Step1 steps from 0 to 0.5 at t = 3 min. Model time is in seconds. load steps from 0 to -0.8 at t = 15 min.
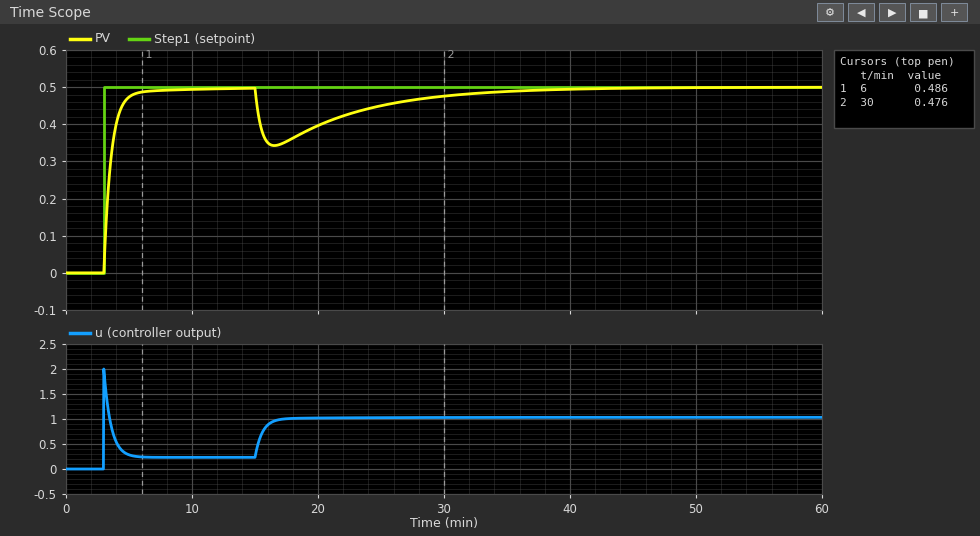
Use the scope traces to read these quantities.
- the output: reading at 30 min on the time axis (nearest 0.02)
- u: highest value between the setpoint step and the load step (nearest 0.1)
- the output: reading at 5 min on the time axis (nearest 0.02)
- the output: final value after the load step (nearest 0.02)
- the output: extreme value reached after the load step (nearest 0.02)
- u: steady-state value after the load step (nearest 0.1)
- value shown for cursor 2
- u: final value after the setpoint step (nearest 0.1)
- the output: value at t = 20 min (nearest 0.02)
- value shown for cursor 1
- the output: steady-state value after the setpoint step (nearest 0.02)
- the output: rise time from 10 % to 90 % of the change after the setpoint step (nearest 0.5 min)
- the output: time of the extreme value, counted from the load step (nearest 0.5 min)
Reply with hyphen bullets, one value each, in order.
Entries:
- 0.48
- 2.0
- 0.48
- 0.50
- 0.34
- 1.0
- 0.476
- 0.2
- 0.40
- 0.486
- 0.50
- 1.5 min
- 1.5 min
